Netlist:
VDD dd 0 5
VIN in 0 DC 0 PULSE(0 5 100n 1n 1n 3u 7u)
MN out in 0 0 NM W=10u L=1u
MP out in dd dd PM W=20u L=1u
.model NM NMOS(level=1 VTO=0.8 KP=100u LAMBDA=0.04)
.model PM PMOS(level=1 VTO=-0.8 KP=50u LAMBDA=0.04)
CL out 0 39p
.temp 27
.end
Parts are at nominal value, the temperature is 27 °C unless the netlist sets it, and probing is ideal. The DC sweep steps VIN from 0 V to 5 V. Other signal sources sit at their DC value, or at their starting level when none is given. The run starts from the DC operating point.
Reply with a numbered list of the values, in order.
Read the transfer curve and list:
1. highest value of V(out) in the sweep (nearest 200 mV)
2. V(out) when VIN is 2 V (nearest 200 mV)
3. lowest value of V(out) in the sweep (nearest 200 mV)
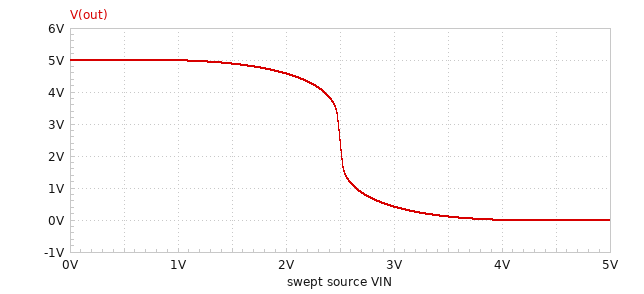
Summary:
1. 5.0 V
2. 4.6 V
3. 0 V
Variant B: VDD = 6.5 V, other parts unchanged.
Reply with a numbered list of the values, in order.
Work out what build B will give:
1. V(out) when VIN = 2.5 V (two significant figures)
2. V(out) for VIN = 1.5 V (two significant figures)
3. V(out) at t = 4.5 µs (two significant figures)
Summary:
1. 5.9 V
2. 6.4 V
3. 6.5 V
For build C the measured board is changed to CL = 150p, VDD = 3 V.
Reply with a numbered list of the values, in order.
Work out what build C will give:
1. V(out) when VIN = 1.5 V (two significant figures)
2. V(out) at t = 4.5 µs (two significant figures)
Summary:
1. 1.5 V
2. 3.0 V
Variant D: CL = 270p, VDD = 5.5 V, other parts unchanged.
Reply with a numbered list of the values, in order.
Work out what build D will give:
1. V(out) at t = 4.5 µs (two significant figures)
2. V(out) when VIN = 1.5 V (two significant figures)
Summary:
1. 5.5 V
2. 5.4 V
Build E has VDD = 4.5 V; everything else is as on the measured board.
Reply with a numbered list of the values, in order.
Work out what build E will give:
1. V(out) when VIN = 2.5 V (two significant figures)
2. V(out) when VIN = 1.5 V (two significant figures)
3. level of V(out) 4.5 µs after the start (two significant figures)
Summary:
1. 580 mV
2. 4.4 V
3. 4.5 V
